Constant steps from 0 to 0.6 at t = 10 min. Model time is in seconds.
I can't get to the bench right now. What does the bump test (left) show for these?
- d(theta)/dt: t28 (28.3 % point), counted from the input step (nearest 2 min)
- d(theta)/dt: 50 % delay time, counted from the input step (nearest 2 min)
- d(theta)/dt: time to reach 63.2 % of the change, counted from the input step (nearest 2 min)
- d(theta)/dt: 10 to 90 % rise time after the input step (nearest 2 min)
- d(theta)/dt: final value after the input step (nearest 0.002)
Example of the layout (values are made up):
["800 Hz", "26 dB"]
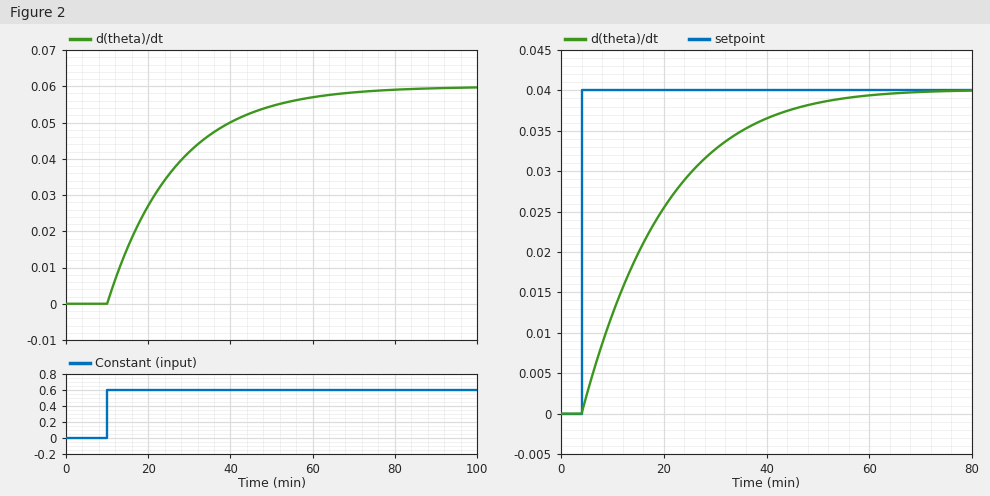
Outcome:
["6 min", "12 min", "16 min", "36 min", "0.060"]
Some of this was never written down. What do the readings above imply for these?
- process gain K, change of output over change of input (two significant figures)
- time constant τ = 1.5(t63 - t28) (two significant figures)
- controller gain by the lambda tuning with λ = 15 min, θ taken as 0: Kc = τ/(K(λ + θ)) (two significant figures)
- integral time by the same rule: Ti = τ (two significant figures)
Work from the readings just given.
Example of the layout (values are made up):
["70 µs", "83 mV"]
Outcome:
["0.10", "15 min", "10", "15 min"]
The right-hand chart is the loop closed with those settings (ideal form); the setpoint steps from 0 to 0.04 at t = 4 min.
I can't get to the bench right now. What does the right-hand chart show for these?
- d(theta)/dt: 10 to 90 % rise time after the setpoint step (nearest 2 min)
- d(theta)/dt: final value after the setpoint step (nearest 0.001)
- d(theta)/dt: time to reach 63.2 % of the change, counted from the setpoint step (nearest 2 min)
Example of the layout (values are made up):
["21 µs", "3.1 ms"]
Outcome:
["32 min", "0.040", "16 min"]
